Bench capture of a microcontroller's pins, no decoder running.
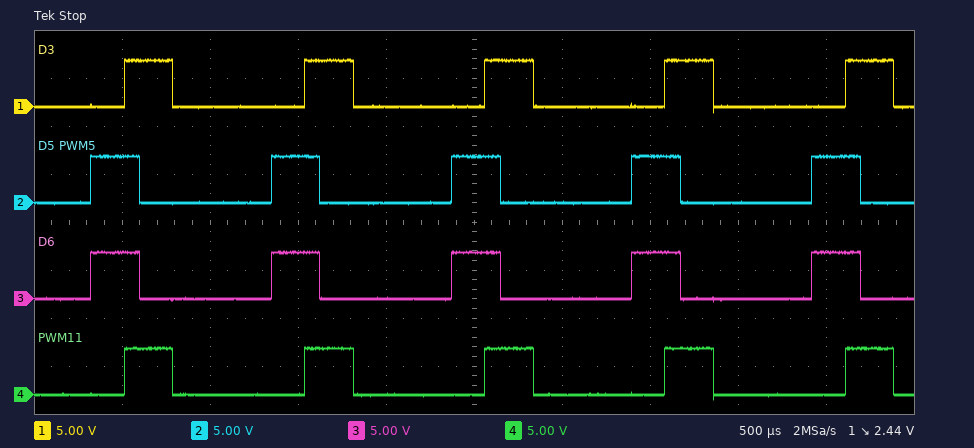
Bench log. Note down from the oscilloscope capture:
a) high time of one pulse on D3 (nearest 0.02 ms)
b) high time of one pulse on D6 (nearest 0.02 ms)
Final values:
0.28 ms
0.28 ms
